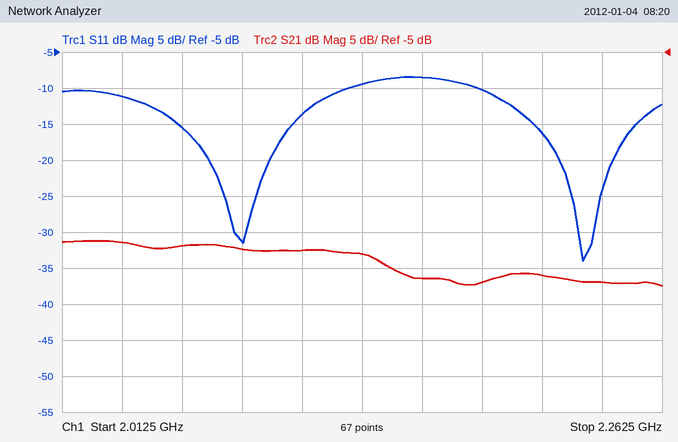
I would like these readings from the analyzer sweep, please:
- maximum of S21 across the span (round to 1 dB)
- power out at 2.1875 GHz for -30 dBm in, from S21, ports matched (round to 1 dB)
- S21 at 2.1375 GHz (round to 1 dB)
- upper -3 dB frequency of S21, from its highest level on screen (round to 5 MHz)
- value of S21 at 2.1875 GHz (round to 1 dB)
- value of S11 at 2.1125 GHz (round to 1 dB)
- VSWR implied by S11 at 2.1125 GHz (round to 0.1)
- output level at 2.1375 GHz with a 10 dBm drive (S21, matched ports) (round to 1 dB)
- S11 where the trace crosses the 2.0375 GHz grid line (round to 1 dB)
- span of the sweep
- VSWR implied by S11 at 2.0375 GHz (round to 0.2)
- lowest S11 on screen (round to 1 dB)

-31 dB
-67 dBm
-33 dB
2.145 GHz
-37 dB
-14 dB
1.5
-23 dBm
-11 dB
250 MHz
1.8
-34 dB
